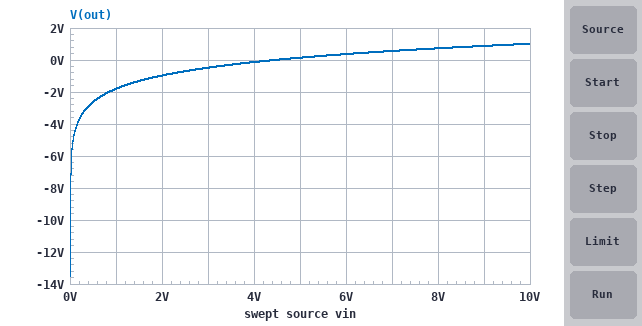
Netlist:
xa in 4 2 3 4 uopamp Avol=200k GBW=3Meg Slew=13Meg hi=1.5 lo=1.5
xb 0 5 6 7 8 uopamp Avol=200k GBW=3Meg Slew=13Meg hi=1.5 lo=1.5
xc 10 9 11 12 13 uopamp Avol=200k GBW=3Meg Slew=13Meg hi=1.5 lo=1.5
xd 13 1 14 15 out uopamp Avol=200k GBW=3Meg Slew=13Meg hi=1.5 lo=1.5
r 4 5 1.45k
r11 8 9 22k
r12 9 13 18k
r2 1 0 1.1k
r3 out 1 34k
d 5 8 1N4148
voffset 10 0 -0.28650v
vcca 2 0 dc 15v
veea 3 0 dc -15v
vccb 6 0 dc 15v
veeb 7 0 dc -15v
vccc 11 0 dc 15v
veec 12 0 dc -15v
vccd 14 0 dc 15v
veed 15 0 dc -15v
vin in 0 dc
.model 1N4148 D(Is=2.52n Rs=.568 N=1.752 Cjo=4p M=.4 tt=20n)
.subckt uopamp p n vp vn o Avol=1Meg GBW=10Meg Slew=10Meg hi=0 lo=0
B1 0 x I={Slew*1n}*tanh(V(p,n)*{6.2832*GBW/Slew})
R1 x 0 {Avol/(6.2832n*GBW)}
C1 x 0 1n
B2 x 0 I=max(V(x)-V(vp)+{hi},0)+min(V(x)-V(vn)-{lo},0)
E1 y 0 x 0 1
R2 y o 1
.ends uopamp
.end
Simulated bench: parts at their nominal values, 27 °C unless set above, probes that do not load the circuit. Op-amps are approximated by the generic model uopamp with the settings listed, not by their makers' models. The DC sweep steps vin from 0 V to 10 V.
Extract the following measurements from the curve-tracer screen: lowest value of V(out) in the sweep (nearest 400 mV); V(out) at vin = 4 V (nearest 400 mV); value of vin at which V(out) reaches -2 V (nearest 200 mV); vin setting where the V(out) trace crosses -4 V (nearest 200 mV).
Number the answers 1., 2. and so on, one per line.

1. -13.6 V
2. 0 V
3. 800 mV
4. 200 mV
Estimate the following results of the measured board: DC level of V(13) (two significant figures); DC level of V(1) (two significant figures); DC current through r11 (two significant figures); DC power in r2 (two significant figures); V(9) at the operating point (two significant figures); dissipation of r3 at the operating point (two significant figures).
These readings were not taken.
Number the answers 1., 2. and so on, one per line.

1. -520 mV
2. -420 mV
3. 13 µA
4. 160 µW
5. -290 mV
6. 5.0 mW
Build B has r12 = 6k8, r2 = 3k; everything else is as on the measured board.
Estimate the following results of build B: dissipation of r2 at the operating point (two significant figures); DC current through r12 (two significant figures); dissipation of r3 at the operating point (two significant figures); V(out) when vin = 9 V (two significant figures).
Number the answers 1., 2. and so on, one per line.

1. 47 µW
2. 13 µA
3. 530 µW
4. -2.1 V
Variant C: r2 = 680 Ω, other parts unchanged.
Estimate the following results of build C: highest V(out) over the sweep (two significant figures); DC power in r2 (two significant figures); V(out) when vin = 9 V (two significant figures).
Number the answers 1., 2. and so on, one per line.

1. 1.6 V
2. 100 µW
3. 1.4 V
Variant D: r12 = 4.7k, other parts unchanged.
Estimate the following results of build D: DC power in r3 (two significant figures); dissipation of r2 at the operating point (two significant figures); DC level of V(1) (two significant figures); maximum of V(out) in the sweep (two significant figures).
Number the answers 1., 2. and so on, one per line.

1. 3.4 mW
2. 110 µW
3. -350 mV
4. -6.5 V
